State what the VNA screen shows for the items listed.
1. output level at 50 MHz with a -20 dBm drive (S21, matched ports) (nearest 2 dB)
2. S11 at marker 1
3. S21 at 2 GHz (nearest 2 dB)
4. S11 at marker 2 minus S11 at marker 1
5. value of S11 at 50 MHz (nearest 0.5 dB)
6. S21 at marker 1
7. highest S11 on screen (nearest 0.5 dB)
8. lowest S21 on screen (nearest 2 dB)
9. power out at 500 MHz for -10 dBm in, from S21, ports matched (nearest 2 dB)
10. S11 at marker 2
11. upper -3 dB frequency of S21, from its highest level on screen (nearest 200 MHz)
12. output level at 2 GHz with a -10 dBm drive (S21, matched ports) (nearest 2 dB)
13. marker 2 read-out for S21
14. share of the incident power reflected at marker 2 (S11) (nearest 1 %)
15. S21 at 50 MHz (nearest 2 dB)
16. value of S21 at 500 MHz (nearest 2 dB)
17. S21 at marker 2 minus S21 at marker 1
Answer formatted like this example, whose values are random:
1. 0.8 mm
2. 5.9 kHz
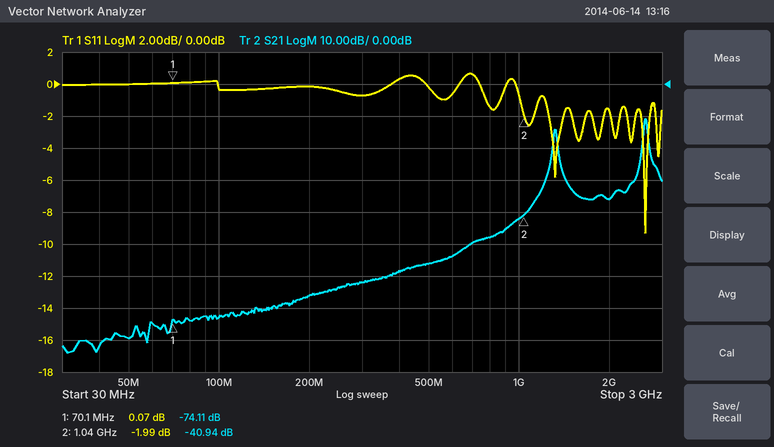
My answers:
1. -100 dBm
2. 0.07 dB
3. -36 dB
4. -2.06 dB
5. 0.0 dB
6. -74.11 dB
7. 0.5 dB
8. -84 dB
9. -66 dBm
10. -1.99 dB
11. 2.6 GHz
12. -46 dBm
13. -40.94 dB
14. 63 %
15. -80 dB
16. -56 dB
17. 33.17 dB
